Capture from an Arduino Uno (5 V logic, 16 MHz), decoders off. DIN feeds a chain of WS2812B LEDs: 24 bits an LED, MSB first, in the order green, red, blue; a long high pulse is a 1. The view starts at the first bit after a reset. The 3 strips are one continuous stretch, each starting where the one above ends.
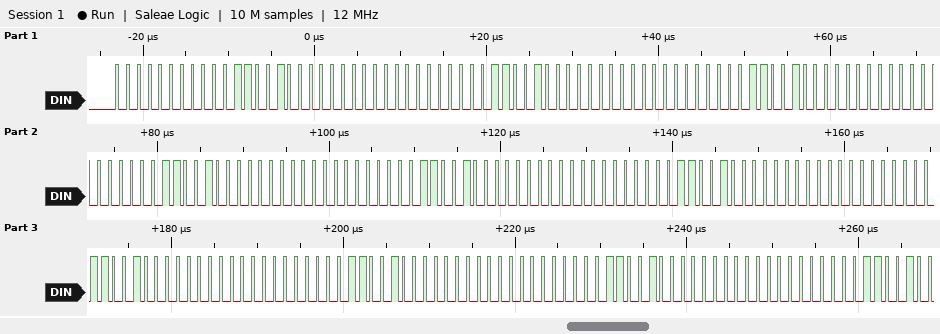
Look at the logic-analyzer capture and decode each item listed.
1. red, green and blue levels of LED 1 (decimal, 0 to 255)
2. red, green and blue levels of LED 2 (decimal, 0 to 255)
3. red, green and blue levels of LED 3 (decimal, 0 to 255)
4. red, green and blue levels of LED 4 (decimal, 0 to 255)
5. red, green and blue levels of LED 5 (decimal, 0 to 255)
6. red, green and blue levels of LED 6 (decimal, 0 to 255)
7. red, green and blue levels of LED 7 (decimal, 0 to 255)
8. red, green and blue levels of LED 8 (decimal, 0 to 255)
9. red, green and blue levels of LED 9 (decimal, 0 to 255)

25, 0, 0
25, 0, 0
25, 0, 0
25, 0, 0
25, 0, 0
25, 0, 0
25, 0, 0
25, 0, 0
25, 0, 0
